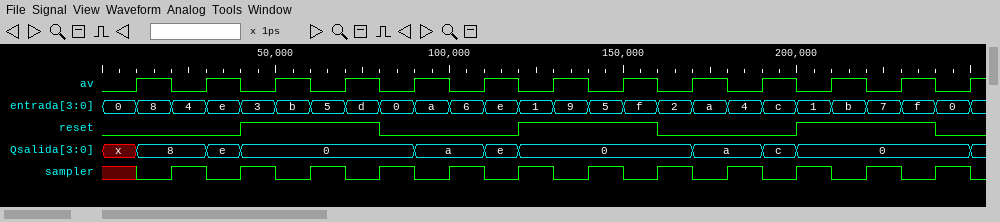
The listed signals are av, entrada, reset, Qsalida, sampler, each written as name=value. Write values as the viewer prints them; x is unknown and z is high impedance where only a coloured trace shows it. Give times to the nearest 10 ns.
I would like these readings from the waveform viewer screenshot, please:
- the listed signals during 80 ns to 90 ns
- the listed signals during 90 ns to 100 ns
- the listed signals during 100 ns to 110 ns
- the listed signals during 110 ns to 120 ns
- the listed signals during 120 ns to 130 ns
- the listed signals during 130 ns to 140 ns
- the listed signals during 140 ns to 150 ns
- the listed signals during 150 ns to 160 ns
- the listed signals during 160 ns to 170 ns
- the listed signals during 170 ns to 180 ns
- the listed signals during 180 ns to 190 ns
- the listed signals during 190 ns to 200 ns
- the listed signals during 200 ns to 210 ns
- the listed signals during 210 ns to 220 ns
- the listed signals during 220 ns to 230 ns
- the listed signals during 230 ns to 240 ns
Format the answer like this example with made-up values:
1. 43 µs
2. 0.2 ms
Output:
1. av=0, entrada=0, reset=0, Qsalida=0, sampler=1
2. av=1, entrada=a, reset=0, Qsalida=a, sampler=0
3. av=0, entrada=6, reset=0, Qsalida=a, sampler=1
4. av=1, entrada=e, reset=0, Qsalida=e, sampler=0
5. av=0, entrada=1, reset=1, Qsalida=0, sampler=1
6. av=1, entrada=9, reset=1, Qsalida=0, sampler=0
7. av=0, entrada=5, reset=1, Qsalida=0, sampler=1
8. av=1, entrada=f, reset=1, Qsalida=0, sampler=0
9. av=0, entrada=2, reset=0, Qsalida=0, sampler=1
10. av=1, entrada=a, reset=0, Qsalida=a, sampler=0
11. av=0, entrada=4, reset=0, Qsalida=a, sampler=1
12. av=1, entrada=c, reset=0, Qsalida=c, sampler=0
13. av=0, entrada=1, reset=1, Qsalida=0, sampler=1
14. av=1, entrada=b, reset=1, Qsalida=0, sampler=0
15. av=0, entrada=7, reset=1, Qsalida=0, sampler=1
16. av=1, entrada=f, reset=1, Qsalida=0, sampler=0
